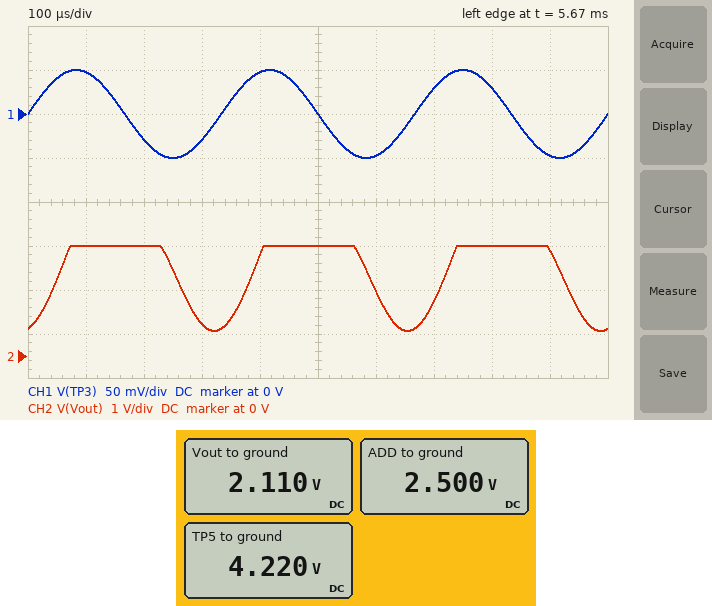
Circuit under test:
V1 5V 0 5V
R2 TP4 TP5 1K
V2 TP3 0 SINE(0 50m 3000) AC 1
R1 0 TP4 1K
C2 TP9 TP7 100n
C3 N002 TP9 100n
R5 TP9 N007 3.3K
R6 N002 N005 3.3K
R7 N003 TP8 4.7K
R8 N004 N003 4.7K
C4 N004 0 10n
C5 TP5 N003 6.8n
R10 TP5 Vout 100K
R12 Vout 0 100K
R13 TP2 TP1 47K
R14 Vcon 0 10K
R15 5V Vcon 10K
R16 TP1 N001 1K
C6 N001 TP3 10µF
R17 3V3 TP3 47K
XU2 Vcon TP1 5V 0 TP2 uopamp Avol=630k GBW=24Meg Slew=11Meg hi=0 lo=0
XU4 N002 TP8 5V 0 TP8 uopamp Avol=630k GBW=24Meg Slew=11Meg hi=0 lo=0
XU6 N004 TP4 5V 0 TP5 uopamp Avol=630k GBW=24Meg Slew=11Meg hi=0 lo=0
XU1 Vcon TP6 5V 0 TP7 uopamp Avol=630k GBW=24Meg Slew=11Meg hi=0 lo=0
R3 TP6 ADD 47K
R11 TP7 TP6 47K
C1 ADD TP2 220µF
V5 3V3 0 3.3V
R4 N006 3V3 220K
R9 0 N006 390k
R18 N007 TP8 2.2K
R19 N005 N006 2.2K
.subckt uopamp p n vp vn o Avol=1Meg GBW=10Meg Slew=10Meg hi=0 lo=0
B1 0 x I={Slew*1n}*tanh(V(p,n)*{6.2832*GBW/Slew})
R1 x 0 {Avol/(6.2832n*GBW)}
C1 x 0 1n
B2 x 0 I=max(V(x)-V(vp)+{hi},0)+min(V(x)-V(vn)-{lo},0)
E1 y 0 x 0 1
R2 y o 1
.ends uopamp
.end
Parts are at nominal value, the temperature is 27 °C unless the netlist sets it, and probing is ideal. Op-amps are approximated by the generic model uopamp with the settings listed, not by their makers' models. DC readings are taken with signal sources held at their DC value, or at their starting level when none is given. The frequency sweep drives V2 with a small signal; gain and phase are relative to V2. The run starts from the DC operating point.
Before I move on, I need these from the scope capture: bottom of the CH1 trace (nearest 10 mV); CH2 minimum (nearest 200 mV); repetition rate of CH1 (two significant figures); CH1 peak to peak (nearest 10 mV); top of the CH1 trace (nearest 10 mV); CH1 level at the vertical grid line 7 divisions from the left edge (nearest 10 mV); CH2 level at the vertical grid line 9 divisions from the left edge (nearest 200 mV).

-50 mV
600 mV
3.0 kHz
100 mV
50 mV
30 mV
2.4 V
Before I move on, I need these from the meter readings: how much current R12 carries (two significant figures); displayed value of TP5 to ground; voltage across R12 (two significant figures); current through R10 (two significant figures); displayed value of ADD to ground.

21 µA
4.220 V
2.1 V
21 µA
2.500 V
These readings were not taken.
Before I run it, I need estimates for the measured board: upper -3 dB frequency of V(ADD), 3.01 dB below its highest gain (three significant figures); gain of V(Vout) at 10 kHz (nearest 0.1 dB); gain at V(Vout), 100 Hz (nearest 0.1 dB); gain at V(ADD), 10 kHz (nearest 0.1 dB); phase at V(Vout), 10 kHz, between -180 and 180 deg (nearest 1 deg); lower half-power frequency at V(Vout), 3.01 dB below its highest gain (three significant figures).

500 kHz
17.5 dB
36.2 dB
33.4 dB
-143 deg
49.3 Hz
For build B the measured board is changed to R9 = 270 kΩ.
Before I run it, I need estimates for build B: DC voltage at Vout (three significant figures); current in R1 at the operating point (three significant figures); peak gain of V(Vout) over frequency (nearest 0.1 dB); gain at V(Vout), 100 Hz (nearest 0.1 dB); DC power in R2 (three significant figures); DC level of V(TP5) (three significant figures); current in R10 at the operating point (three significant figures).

1.82 V
1.82 mA
41.0 dB
36.6 dB
3.31 mW
3.64 V
18.2 µA
